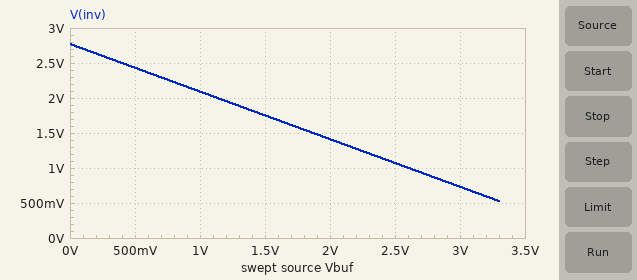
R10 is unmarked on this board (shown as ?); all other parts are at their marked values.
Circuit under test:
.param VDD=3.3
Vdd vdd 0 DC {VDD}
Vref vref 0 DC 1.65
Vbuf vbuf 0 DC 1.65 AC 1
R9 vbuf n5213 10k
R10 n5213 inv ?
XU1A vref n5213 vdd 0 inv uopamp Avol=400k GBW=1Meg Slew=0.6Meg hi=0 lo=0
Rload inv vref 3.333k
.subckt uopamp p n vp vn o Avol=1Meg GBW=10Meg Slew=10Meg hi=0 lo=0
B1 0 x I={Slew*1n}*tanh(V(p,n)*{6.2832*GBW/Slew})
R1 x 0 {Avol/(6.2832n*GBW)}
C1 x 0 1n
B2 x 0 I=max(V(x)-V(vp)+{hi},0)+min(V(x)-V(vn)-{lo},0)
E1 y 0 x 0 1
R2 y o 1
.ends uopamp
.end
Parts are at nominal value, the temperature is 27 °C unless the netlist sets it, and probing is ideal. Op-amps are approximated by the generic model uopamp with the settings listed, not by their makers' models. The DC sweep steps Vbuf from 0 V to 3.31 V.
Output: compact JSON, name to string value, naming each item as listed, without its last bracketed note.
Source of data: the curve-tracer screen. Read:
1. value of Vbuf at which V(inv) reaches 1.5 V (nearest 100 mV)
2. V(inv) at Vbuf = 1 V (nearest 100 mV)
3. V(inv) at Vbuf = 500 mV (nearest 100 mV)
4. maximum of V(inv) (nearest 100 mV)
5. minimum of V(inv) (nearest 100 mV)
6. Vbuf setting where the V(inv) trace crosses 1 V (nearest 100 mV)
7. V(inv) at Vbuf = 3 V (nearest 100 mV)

{"value of Vbuf at which V(inv) reaches 1.5 V": "1.9 V", "V(inv) at Vbuf = 1 V": "2.1 V", "V(inv) at Vbuf = 500 mV": "2.4 V", "maximum of V(inv)": "2.8 V", "minimum of V(inv)": "500 mV", "Vbuf setting where the V(inv) trace crosses 1 V": "2.6 V", "V(inv) at Vbuf = 3 V": "700 mV"}
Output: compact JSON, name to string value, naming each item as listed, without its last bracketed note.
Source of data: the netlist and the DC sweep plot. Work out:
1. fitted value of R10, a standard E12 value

{"fitted value of R10, a standard E12 value": "6.8 kΩ"}
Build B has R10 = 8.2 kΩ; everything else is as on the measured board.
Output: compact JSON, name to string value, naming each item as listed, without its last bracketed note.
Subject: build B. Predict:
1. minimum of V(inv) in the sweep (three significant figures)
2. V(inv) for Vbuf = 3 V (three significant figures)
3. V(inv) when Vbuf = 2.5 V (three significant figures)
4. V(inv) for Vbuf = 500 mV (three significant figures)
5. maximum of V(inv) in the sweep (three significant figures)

{"minimum of V(inv) in the sweep": "289 mV", "V(inv) for Vbuf = 3 V": "543 mV", "V(inv) when Vbuf = 2.5 V": "953 mV", "V(inv) for Vbuf = 500 mV": "2.59 V", "maximum of V(inv) in the sweep": "3.00 V"}
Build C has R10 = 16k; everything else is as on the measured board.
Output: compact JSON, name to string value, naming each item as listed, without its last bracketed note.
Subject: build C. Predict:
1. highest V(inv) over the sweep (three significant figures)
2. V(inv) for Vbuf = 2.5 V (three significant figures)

{"highest V(inv) over the sweep": "3.30 V", "V(inv) for Vbuf = 2.5 V": "290 mV"}
